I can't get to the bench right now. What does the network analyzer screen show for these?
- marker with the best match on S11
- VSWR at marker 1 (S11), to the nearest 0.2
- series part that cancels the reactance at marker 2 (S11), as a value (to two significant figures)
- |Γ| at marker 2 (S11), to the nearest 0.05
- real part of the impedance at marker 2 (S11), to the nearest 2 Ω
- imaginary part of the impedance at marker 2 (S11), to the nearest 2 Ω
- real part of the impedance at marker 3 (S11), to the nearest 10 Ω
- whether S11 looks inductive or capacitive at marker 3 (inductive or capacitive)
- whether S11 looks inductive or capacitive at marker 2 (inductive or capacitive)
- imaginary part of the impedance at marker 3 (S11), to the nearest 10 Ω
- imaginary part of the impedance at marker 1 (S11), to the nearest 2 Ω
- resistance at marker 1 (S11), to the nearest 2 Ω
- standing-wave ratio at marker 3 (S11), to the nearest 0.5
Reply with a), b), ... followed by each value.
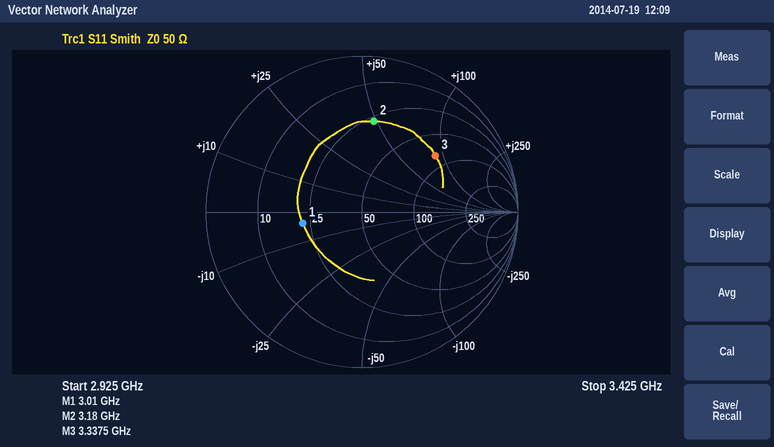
a) marker 1
b) 2.2
c) 1.0 pF
d) 0.60
e) 28 Ω
f) +48 Ω
g) 80 Ω
h) inductive
i) inductive
j) +90 Ω
k) -4 Ω
l) 22 Ω
m) 4.0
